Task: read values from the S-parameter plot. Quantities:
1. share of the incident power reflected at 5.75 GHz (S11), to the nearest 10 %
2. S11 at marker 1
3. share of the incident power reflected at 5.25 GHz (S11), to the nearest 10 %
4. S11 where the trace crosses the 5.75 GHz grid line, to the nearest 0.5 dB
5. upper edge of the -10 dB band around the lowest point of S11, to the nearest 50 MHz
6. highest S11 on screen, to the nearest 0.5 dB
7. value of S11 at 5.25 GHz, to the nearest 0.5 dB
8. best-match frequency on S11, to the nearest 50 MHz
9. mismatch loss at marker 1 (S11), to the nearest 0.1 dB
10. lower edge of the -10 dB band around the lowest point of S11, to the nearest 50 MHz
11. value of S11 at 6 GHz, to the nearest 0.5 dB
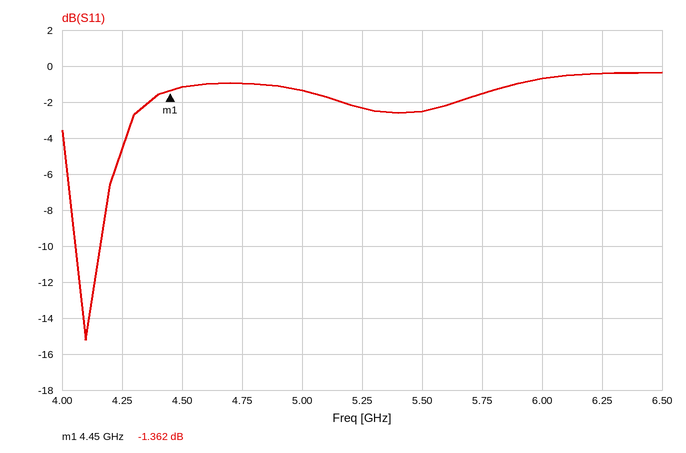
70 %
-1.362 dB
60 %
-1.5 dB
4.15 GHz
-0.5 dB
-2.5 dB
4.10 GHz
5.7 dB
4.05 GHz
-0.5 dB
